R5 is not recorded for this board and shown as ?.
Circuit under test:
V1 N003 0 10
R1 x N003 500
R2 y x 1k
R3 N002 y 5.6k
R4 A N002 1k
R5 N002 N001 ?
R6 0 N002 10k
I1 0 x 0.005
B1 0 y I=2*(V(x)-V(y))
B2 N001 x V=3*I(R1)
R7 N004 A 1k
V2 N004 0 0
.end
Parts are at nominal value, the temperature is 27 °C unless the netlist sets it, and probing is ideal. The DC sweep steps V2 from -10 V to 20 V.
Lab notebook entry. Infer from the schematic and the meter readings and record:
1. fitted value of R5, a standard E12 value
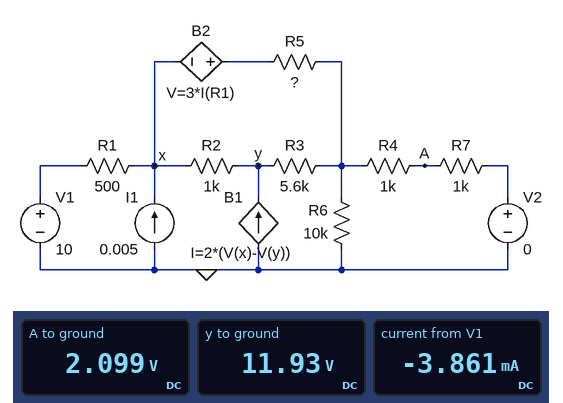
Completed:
6.8 kΩ
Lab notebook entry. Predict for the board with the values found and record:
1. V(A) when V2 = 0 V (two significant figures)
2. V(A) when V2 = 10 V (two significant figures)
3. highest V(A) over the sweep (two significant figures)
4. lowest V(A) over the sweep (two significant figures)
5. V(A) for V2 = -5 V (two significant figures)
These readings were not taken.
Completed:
2.1 V
9.9 V
18 V
-5.7 V
-1.8 V
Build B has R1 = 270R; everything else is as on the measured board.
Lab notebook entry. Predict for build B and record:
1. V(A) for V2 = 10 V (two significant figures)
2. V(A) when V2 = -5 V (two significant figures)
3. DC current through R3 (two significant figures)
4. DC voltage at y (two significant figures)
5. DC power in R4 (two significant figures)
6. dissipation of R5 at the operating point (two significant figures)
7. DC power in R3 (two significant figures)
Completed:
9.7 V
-1.9 V
1.3 mA
11 V
3.8 mW
7.6 mW
9.2 mW
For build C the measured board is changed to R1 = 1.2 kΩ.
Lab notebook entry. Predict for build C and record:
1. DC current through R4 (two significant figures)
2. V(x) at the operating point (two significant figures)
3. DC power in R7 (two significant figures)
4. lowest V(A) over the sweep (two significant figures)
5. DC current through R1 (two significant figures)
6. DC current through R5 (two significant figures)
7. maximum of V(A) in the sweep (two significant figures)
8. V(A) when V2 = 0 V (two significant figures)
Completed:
2.5 mA
14 V
6.4 mW
-5.3 V
3.6 mA
1.4 mA
18 V
2.5 V
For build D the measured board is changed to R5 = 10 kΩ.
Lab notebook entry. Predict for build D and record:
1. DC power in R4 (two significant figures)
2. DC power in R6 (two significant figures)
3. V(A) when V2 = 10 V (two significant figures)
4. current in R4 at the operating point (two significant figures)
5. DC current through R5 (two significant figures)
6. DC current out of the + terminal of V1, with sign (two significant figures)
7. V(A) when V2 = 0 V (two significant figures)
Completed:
3.7 mW
1.5 mW
9.8 V
1.9 mA
830 µA
-4.2 mA
1.9 V
